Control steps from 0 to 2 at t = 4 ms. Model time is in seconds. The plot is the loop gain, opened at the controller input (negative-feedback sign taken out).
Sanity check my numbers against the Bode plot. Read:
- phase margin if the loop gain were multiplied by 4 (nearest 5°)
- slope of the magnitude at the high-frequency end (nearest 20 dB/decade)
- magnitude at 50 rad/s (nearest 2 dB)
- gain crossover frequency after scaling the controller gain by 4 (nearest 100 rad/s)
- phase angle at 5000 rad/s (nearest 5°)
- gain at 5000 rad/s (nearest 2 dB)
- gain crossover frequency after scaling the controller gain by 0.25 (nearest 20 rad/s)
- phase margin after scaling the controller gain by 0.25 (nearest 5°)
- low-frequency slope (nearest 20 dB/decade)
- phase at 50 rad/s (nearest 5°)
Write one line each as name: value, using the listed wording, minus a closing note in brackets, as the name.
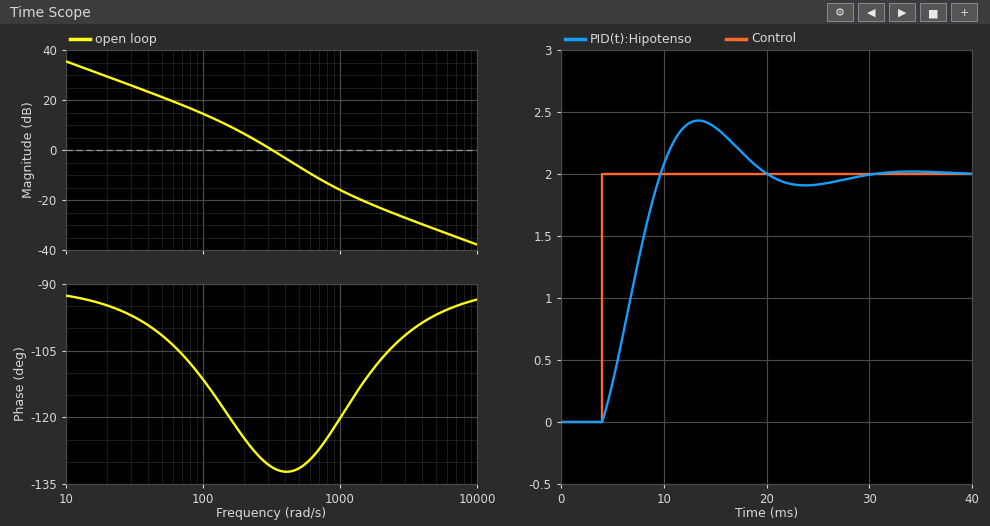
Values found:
phase margin if the loop gain were multiplied by 4: 55°
slope of the magnitude at the high-frequency end: -20 dB/decade
magnitude at 50 rad/s: 22 dB
gain crossover frequency after scaling the controller gain by 4: 700 rad/s
phase angle at 5000 rad/s: -95°
gain at 5000 rad/s: -32 dB
gain crossover frequency after scaling the controller gain by 0.25: 120 rad/s
phase margin after scaling the controller gain by 0.25: 65°
low-frequency slope: -20 dB/decade
phase at 50 rad/s: -100°
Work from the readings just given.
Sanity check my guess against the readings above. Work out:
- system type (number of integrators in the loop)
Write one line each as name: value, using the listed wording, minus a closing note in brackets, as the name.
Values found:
system type: 1
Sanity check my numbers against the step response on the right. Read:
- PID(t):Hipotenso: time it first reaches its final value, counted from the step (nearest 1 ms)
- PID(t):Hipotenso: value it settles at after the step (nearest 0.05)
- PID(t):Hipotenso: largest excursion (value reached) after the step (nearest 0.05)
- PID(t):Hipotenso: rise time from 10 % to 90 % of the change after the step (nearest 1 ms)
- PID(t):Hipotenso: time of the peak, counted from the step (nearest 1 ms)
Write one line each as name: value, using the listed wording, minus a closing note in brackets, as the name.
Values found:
PID(t):Hipotenso: time it first reaches its final value, counted from the step: 6 ms
PID(t):Hipotenso: value it settles at after the step: 2.00
PID(t):Hipotenso: largest excursion (value reached) after the step: 2.45
PID(t):Hipotenso: rise time from 10 % to 90 % of the change after the step: 4 ms
PID(t):Hipotenso: time of the peak, counted from the step: 9 ms
